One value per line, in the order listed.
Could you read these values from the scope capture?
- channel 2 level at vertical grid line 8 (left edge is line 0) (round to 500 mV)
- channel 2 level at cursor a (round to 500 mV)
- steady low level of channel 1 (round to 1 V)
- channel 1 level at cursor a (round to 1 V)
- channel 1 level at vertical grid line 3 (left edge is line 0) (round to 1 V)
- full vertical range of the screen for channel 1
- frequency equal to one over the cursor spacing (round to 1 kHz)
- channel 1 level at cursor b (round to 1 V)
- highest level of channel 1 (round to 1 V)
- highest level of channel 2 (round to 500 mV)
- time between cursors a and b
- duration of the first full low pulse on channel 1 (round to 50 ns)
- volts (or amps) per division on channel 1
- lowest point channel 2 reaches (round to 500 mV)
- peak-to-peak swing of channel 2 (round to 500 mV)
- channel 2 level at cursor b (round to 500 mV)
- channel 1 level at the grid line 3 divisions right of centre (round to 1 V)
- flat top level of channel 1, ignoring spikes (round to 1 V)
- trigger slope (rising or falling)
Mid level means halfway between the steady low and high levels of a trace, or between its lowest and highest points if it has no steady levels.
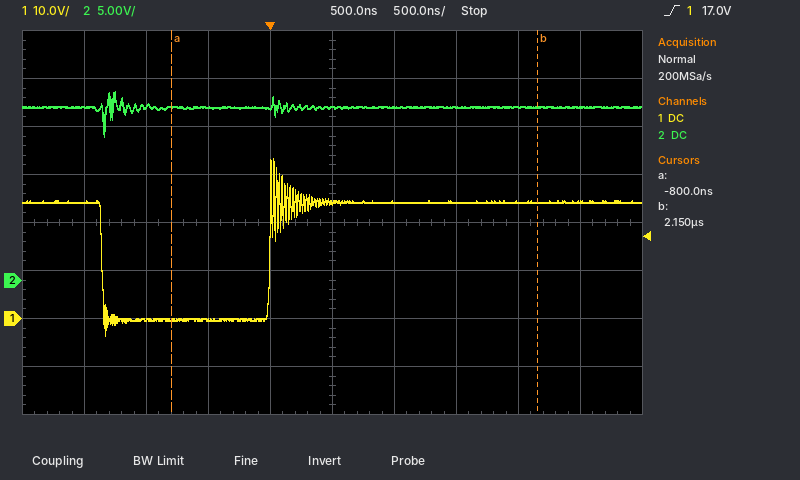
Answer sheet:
18.0 V
18.0 V
0 V
0 V
0 V
80 V
339 kHz
24 V
33 V
19.5 V
2.95 µs
1.35 µs
10 V
15.0 V
4.5 V
18.0 V
24 V
24 V
rising
